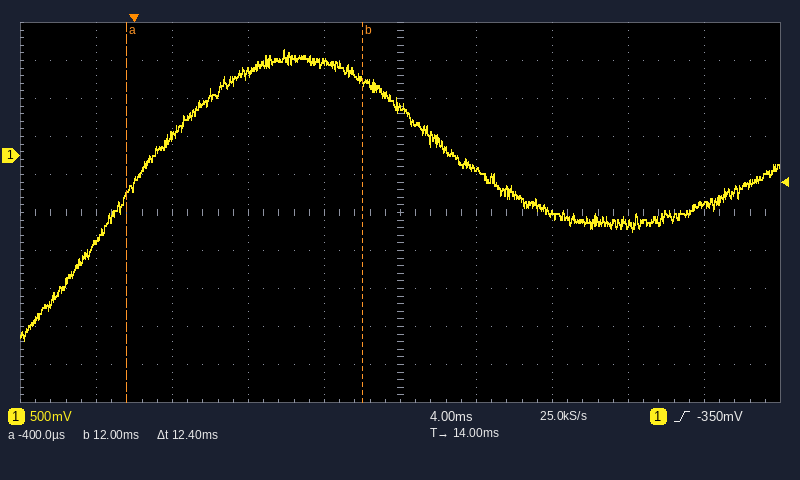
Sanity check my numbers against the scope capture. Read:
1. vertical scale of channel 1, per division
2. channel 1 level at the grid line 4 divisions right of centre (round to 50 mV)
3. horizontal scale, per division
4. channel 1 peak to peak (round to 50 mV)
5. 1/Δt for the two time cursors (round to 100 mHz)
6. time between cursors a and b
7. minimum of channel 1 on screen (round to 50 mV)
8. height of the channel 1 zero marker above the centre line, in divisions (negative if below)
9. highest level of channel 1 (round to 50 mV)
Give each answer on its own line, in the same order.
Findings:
500 mV
-650 mV
4 ms
3.85 V
80.6 Hz
12.4 ms
-2.45 V
+1.5 div
1.40 V
